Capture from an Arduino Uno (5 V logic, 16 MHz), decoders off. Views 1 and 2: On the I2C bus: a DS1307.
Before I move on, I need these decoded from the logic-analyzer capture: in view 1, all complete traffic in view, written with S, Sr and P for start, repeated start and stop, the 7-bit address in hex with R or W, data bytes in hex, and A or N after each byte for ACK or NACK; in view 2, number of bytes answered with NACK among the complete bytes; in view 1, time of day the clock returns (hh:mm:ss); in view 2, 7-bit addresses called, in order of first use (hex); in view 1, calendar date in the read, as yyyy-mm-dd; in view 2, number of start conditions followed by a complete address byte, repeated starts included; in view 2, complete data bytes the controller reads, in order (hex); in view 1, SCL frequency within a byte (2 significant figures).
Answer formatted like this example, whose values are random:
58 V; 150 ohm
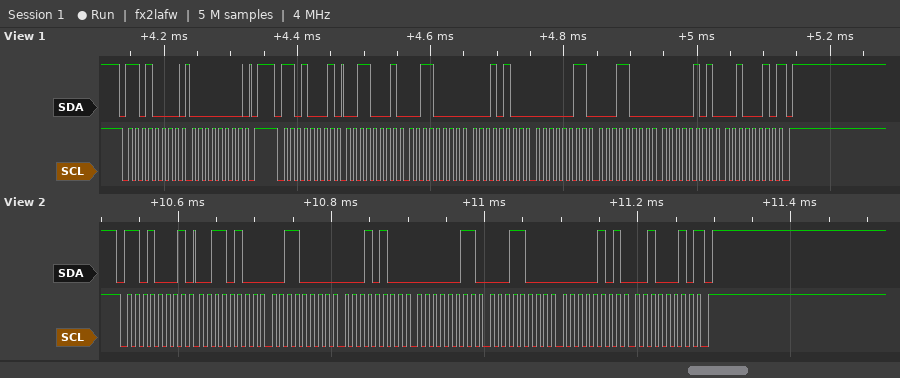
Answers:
S 68W A 00 A P S 68R A 31 A 30 A 14 A 03 A 18 A 05 A 22 N P; 1; 14:30:31; 0x68; 2022-05-18; 1; 34 30 14 03 18 05 22; 100 kHz
